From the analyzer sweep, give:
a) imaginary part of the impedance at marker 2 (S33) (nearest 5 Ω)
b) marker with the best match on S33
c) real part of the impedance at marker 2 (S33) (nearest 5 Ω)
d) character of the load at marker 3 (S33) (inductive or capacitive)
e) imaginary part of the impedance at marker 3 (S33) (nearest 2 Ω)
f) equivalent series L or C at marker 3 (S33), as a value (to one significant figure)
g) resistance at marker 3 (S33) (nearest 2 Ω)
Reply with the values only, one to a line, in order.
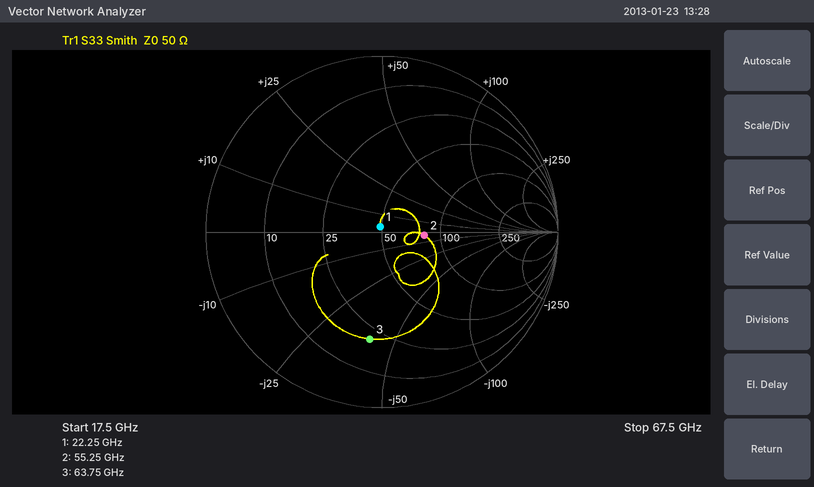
-5 Ω
marker 1
80 Ω
capacitive
-40 Ω
60 fF
20 Ω
